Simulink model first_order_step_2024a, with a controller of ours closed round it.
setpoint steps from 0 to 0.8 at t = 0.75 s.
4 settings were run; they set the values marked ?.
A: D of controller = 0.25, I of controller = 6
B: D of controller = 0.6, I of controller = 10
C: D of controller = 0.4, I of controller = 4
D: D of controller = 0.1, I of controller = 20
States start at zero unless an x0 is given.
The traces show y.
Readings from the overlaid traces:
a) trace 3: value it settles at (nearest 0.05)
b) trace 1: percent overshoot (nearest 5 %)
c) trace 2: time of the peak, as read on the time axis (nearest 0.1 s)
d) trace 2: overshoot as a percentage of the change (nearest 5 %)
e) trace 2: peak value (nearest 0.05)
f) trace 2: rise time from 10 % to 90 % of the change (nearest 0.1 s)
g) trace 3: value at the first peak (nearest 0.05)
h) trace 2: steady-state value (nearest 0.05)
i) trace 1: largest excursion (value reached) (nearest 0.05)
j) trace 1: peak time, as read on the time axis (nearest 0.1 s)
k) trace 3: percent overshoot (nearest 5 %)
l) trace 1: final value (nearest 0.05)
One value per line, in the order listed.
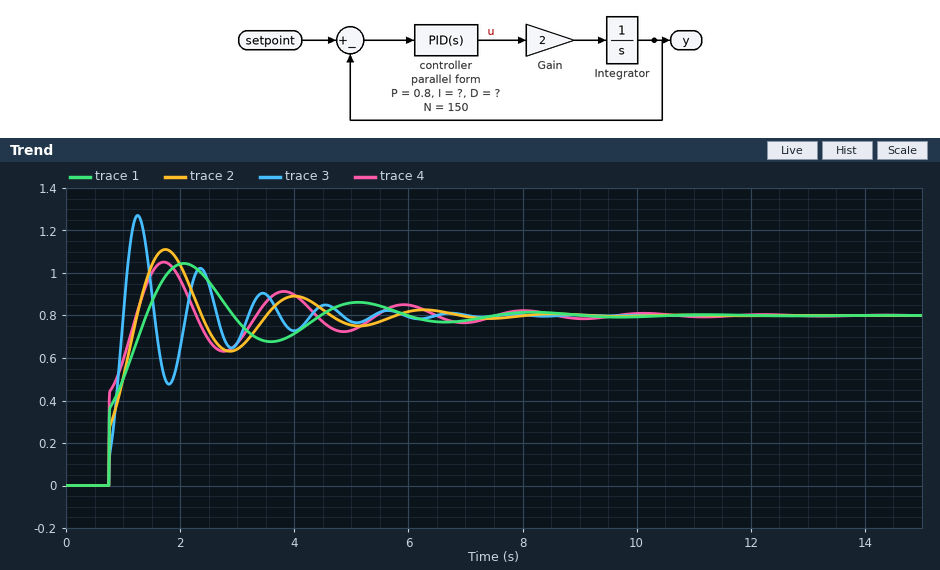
0.80
30 %
1.7 s
40 %
1.10
0.4 s
1.25
0.80
1.05
2.1 s
60 %
0.80
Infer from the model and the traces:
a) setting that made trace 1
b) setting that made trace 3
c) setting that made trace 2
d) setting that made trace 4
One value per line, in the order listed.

C
D
A
B
